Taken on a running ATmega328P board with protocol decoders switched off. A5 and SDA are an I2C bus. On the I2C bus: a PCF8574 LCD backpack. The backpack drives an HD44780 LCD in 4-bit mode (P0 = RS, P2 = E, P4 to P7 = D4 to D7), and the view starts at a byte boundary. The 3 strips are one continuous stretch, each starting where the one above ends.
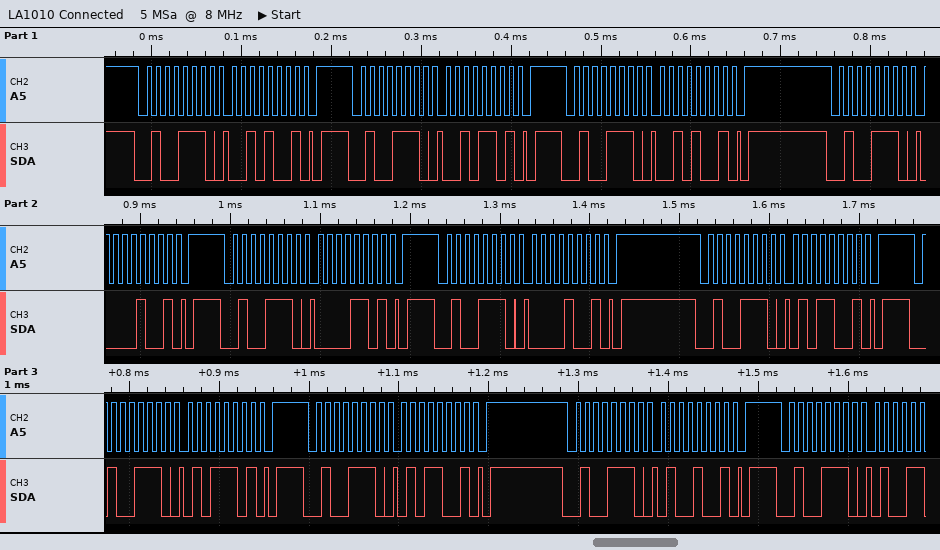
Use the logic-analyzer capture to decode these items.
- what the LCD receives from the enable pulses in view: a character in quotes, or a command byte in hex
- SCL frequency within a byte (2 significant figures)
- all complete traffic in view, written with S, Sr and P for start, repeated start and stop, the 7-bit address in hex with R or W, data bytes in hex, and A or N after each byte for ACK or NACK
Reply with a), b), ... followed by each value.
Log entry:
a) ' '
b) 100 kHz
c) S 27W A 29 A P S 27W A 2D A P S 27W A 29 A P S 27W A 09 A P S 27W A 0D A P S 27W A 09 A P S 27W A 59 A P S 27W A 5D A P S 27W A 59 A P S 27W A 49 A P S 27W A
